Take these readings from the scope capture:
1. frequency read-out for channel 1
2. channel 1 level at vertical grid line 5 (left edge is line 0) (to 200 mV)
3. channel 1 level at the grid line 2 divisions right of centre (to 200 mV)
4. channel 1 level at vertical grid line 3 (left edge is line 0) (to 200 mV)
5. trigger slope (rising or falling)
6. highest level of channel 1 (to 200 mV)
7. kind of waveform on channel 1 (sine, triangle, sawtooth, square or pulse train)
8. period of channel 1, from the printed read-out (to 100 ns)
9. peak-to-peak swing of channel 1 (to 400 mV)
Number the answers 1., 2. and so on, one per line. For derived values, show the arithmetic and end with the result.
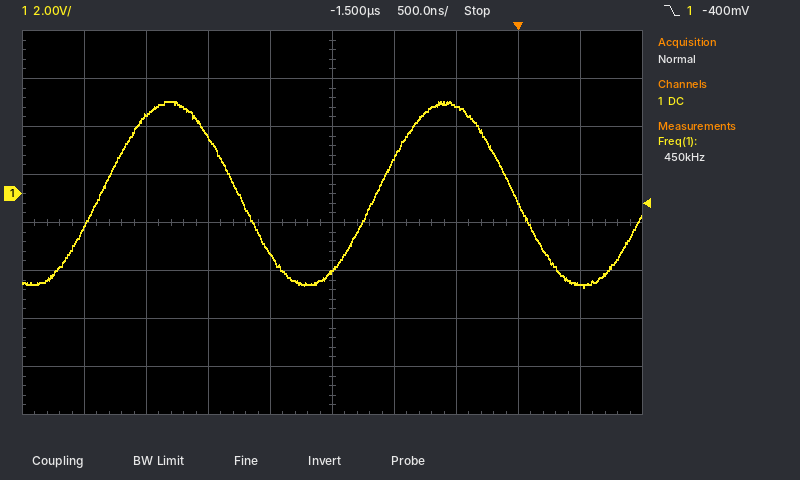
1. 450 kHz
2. -3.2 V
3. 3.6 V
4. 2.4 V
5. falling
6. 3.8 V
7. sine
8. 1 / 450 kHz ≈ 2.2 µs
9. 7.6 V
